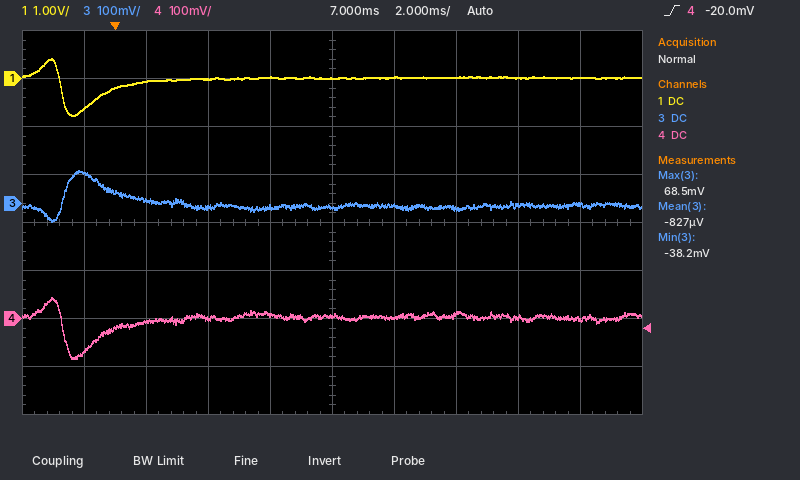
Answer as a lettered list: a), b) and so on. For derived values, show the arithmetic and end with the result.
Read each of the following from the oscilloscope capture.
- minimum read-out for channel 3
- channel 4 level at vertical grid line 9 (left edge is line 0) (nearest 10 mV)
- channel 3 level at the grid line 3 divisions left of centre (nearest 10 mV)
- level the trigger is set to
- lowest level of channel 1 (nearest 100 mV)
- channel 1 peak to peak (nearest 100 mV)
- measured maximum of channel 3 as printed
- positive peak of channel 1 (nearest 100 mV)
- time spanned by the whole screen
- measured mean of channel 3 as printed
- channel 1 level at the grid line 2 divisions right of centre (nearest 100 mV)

a) -38.2 mV
b) 0 mV
c) 10 mV
d) -20.0 mV
e) -800 mV
f) 400 mV − (-800 mV) = 1.2 V
g) 68.5 mV
h) 400 mV
i) 20 ms
j) -827 µV
k) 0.0 V
